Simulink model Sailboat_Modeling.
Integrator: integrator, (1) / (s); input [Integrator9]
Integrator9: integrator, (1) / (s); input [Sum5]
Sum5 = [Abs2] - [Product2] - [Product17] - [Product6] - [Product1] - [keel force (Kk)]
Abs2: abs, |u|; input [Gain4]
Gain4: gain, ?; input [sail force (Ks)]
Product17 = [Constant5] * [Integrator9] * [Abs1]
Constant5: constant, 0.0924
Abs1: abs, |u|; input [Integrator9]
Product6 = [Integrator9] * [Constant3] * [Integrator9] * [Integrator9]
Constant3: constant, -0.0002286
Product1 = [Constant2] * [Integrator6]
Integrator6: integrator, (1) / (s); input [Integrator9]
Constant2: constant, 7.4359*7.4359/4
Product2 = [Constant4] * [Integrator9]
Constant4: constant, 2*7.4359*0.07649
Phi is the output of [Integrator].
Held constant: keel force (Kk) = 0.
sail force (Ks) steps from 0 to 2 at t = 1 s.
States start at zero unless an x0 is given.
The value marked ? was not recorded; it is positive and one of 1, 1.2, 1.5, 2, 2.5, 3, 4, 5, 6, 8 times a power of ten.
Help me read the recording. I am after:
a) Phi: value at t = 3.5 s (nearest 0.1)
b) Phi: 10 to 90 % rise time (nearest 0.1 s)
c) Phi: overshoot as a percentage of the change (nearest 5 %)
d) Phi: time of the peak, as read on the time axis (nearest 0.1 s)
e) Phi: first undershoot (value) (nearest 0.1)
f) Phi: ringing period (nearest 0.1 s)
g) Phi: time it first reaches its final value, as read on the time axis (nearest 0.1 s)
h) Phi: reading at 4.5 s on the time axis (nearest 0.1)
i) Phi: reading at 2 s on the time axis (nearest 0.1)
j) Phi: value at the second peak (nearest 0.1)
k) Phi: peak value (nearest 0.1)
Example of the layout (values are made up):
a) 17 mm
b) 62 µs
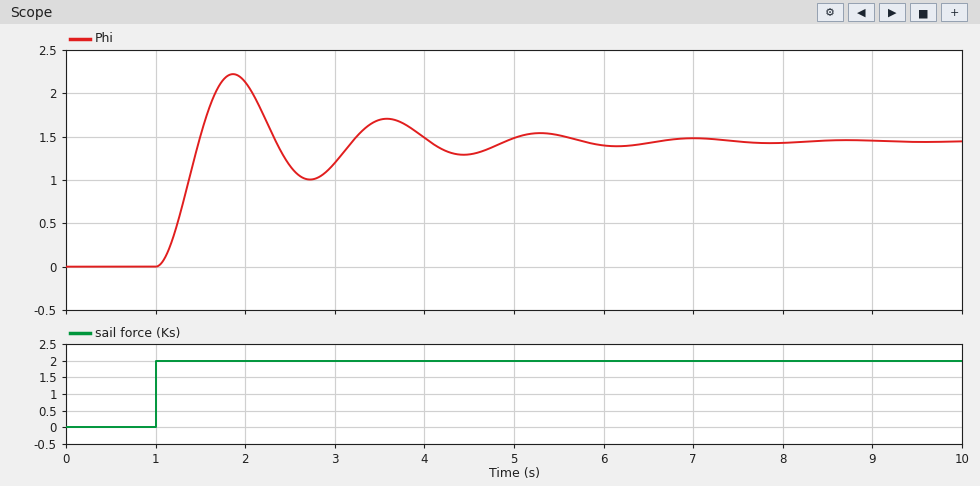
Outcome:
a) 1.7
b) 0.3 s
c) 55 %
d) 1.9 s
e) 1.0
f) 1.7 s
g) 1.5 s
h) 1.3
i) 2.1
j) 1.7
k) 2.2
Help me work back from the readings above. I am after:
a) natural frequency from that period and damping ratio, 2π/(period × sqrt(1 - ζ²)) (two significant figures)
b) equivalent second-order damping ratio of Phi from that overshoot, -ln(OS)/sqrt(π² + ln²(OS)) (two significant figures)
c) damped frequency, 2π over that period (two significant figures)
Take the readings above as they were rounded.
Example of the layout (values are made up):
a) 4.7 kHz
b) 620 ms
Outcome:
a) 3.8 rad/s
b) 0.19
c) 3.7 rad/s
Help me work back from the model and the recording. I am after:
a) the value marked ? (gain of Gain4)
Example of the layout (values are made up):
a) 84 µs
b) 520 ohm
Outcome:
a) 10
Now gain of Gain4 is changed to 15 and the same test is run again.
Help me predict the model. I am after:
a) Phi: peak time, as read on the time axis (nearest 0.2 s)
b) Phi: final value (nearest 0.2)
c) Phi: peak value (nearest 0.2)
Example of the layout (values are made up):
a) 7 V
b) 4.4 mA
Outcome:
a) 1.8 s
b) 2.2
c) 3.2
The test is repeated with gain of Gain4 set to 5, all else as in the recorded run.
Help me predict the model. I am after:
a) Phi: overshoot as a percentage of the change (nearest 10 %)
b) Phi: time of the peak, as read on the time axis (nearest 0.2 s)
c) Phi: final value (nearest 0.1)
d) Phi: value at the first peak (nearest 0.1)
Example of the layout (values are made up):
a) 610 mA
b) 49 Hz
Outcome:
a) 60 %
b) 1.8 s
c) 0.7
d) 1.1
